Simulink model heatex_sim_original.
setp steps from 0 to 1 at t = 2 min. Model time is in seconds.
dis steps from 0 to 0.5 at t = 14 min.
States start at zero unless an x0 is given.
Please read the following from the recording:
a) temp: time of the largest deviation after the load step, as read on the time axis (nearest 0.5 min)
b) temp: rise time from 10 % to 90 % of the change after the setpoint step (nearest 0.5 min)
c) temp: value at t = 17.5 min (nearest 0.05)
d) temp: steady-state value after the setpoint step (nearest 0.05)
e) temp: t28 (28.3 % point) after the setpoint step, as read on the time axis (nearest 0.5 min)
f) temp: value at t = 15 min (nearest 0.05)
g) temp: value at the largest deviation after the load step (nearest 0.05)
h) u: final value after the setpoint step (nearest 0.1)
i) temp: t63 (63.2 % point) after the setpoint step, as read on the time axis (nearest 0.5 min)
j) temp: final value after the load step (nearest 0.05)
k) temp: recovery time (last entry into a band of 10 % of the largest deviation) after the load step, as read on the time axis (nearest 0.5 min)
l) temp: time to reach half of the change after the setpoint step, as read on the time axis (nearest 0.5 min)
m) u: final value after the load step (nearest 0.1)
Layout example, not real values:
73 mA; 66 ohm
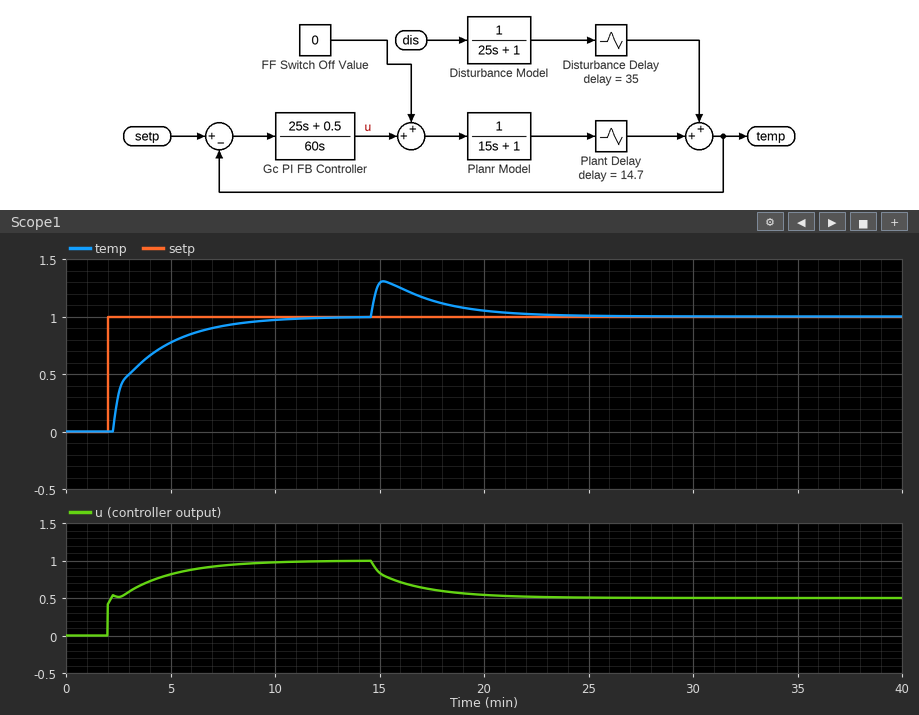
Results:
15.0 min; 4.5 min; 1.15; 1.00; 2.5 min; 1.30; 1.30; 1.0; 4.0 min; 1.00; 21.0 min; 3.0 min; 0.5
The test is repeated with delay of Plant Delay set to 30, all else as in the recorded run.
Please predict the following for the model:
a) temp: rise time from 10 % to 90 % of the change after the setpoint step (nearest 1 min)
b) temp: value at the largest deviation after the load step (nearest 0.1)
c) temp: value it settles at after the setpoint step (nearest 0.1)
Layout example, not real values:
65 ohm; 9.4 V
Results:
4 min; 1.4; 1.0
